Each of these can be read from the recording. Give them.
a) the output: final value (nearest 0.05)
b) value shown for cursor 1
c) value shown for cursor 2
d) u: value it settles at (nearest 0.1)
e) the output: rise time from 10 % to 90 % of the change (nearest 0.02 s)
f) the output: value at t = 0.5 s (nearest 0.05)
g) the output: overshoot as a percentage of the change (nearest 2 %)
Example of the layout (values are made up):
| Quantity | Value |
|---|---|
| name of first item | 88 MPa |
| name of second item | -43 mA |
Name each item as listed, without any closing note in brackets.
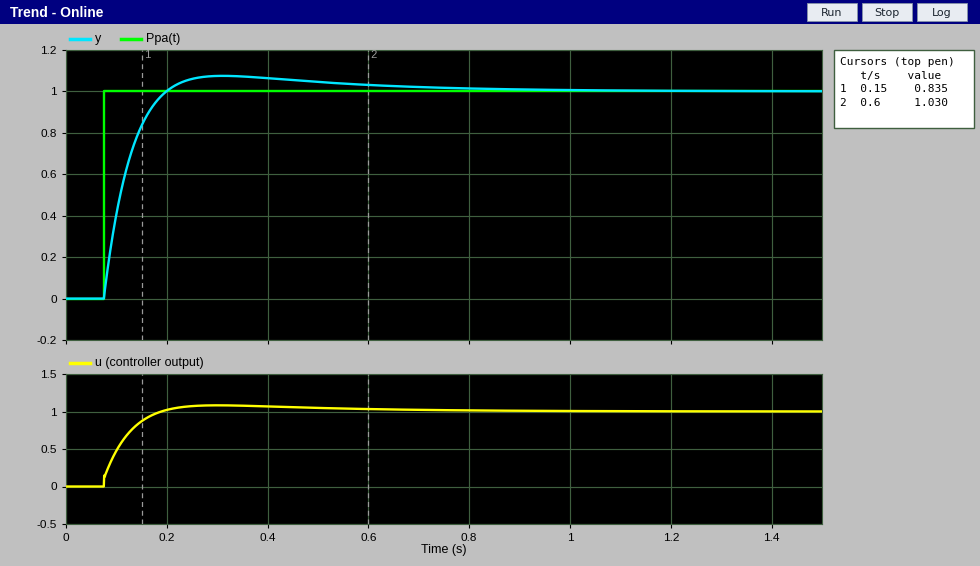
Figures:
| Quantity | Value |
|---|---|
| the output: final value | 1.00 |
| value shown for cursor 1 | 0.835 |
| value shown for cursor 2 | 1.030 |
| u: value it settles at | 1.0 |
| the output: rise time from 10 % to 90 % of the change | 0.08 s |
| the output: value at t = 0.5 s | 1.05 |
| the output: overshoot as a percentage of the change | 8 % |
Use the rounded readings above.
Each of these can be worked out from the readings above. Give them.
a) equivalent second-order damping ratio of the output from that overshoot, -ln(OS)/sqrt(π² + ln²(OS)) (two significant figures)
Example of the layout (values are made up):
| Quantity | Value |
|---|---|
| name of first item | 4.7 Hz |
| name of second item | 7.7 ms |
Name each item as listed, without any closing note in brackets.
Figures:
| Quantity | Value |
|---|---|
| equivalent second-order damping ratio of the output from that overshoot, -ln(OS)/sqrt(π² + ln²(OS)) | 0.63 |
